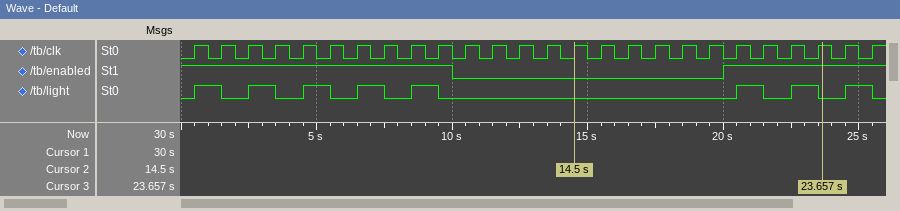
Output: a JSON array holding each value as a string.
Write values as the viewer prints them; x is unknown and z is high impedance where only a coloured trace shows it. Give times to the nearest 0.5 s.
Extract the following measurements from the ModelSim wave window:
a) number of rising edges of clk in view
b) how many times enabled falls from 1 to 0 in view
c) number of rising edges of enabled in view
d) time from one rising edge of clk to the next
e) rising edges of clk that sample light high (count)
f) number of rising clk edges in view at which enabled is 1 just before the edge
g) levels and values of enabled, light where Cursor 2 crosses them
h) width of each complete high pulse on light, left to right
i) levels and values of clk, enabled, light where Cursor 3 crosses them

["26", "1", "1", "1 s", "8", "16", "enabled=0, light=0", "1 s, 1 s, 1 s, 1 s, 1 s, 1 s, 1 s, 1 s", "clk=1, enabled=1, light=0"]
